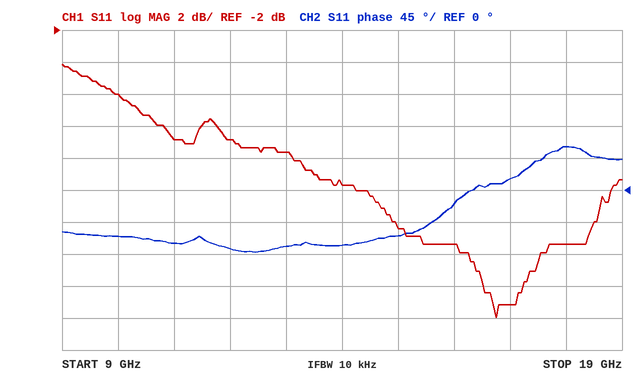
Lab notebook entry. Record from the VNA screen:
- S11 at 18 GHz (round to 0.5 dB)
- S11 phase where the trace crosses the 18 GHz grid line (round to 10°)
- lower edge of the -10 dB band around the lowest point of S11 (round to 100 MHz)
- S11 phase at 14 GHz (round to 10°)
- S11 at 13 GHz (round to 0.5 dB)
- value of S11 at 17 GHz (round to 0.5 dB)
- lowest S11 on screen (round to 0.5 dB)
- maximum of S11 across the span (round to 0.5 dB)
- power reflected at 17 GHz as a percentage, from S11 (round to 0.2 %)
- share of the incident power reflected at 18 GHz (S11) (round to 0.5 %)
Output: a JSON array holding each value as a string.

["-15.5 dB", "60°", "13.1 GHz", "-80°", "-9.5 dB", "-19.0 dB", "-20.0 dB", "-4.0 dB", "1.2 %", "3.0 %"]
